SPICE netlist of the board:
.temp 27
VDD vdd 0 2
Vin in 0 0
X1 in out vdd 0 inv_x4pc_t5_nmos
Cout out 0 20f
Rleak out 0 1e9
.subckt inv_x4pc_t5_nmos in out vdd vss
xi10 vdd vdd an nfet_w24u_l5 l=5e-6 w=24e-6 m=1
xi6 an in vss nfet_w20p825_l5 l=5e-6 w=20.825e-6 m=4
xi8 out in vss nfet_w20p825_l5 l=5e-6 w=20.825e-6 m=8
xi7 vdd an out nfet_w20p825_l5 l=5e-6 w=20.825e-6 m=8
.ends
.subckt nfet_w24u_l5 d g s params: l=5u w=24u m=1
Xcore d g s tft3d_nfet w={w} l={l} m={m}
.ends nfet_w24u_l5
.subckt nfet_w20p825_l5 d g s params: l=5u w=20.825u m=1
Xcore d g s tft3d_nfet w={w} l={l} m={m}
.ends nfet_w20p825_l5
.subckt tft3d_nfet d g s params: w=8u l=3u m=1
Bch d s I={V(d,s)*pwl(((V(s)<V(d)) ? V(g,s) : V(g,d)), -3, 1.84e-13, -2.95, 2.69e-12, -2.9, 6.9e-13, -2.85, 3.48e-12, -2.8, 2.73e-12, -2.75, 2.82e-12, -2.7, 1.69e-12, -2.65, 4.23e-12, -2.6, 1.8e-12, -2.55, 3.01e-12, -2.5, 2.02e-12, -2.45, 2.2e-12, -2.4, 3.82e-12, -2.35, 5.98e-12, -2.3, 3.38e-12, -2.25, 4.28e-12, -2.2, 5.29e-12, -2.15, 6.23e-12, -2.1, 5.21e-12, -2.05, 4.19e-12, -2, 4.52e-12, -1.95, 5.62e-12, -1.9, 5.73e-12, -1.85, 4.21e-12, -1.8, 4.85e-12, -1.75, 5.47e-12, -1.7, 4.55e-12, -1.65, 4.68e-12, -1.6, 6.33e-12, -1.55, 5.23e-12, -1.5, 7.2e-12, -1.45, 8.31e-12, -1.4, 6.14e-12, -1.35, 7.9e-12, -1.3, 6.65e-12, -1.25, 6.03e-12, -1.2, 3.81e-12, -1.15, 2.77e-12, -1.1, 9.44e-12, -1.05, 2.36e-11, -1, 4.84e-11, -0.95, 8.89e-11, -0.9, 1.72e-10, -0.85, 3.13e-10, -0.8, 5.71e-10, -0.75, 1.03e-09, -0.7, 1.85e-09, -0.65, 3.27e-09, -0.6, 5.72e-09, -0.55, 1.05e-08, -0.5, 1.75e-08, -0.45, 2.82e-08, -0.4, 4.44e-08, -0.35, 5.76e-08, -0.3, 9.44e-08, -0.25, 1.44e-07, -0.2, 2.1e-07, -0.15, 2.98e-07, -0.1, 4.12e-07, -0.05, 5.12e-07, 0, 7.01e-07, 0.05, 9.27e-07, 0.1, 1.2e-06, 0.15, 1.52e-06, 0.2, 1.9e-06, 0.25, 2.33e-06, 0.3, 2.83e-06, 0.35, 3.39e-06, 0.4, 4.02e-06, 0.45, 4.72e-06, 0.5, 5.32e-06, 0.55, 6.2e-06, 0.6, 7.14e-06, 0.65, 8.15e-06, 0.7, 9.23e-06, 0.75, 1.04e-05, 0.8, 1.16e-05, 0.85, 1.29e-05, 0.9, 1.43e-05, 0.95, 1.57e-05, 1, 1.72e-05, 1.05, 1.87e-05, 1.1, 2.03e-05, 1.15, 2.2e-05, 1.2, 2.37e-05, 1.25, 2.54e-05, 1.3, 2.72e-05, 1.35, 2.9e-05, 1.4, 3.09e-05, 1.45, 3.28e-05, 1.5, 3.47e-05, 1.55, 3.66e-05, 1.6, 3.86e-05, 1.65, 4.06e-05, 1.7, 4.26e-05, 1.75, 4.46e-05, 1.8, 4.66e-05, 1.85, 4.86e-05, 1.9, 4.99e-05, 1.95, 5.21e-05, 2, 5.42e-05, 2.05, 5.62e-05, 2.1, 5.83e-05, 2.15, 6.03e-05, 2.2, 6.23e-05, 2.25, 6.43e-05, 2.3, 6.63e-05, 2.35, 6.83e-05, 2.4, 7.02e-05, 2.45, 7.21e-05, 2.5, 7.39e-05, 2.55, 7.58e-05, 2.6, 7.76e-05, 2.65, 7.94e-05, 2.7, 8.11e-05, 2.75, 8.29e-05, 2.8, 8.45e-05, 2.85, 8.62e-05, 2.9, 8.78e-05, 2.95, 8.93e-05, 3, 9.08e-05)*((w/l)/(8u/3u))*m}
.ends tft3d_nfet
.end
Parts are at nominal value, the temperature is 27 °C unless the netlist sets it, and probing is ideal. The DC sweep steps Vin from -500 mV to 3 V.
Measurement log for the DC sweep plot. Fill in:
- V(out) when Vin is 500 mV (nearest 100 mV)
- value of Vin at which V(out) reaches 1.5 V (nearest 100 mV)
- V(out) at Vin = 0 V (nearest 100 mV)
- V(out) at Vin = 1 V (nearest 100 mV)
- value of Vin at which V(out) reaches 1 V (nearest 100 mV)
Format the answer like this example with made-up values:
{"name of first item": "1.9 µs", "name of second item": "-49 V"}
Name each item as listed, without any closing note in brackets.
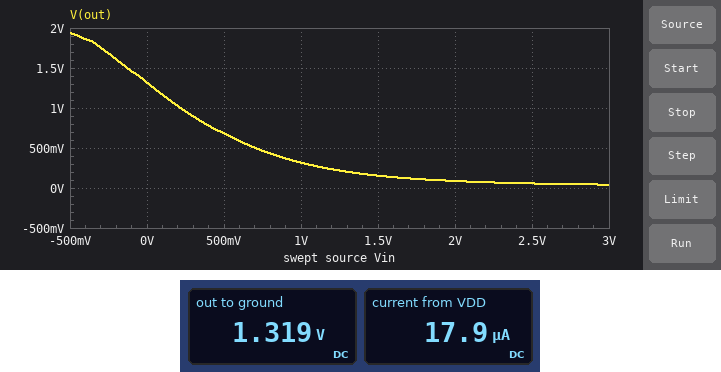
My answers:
{"V(out) when Vin is 500 mV": "700 mV", "value of Vin at which V(out) reaches 1.5 V": "-100 mV", "V(out) at Vin = 0 V": "1.3 V", "V(out) at Vin = 1 V": "300 mV", "value of Vin at which V(out) reaches 1 V": "200 mV"}
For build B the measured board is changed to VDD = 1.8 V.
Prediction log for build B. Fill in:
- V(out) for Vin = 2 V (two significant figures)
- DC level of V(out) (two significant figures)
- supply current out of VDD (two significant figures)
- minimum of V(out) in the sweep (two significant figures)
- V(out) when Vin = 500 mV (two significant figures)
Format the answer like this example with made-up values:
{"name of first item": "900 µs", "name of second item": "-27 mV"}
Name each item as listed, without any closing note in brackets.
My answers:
{"V(out) for Vin = 2 V": "66 mV", "DC level of V(out)": "1.2 V", "supply current out of VDD": "16 µA", "minimum of V(out) in the sweep": "32 mV", "V(out) when Vin = 500 mV": "570 mV"}
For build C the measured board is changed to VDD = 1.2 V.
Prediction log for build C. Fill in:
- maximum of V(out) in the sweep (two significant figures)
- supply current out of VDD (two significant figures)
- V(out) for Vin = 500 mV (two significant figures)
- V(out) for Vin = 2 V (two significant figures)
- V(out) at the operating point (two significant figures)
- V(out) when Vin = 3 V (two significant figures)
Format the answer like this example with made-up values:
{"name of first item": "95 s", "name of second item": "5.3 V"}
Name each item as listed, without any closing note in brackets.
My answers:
{"maximum of V(out) in the sweep": "1.2 V", "supply current out of VDD": "9.6 µA", "V(out) for Vin = 500 mV": "280 mV", "V(out) for Vin = 2 V": "25 mV", "V(out) at the operating point": "710 mV", "V(out) when Vin = 3 V": "13 mV"}
